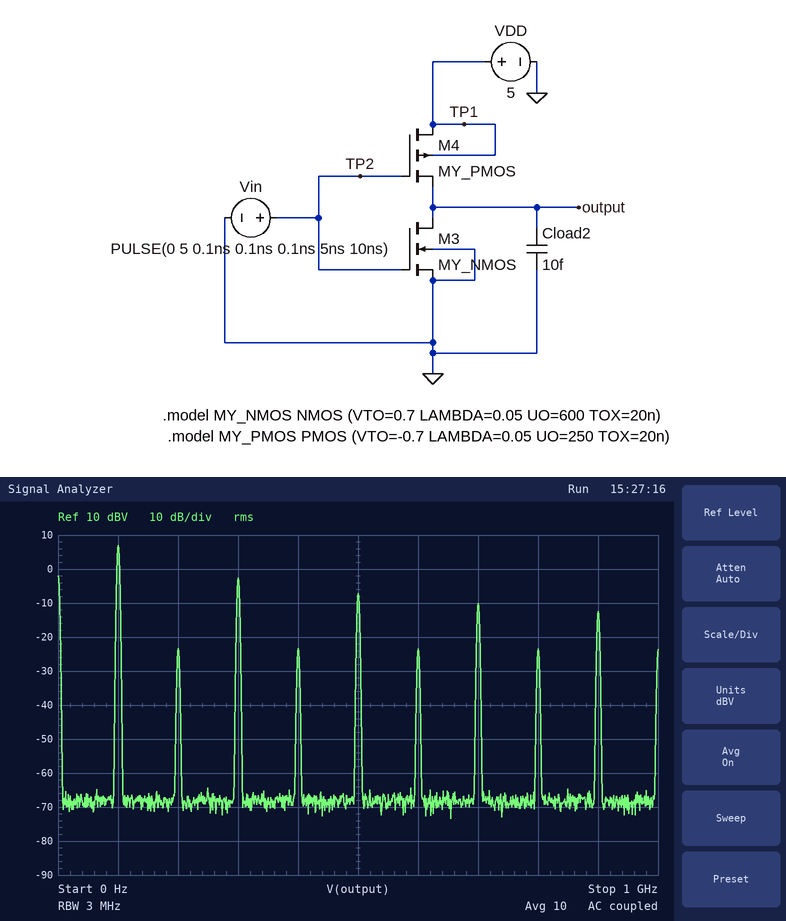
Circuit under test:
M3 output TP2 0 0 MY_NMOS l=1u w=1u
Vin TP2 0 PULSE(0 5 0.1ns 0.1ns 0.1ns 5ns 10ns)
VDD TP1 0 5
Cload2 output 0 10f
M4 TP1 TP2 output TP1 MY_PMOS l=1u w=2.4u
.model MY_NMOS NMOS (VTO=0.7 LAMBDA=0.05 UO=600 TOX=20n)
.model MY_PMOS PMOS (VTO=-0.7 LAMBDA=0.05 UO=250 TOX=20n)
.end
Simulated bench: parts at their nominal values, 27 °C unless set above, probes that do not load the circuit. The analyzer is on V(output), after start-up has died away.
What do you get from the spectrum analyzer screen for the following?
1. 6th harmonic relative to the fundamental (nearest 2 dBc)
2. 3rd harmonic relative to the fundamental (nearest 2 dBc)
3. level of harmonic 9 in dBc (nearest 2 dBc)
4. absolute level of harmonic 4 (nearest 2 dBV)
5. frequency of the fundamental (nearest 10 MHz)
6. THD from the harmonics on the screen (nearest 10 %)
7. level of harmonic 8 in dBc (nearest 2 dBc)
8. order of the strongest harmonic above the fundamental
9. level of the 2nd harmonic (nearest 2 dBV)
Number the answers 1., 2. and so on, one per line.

1. -30 dBc
2. -10 dBc
3. -20 dBc
4. -24 dBV
5. 100 MHz
6. 40 %
7. -30 dBc
8. 3
9. -24 dBV
